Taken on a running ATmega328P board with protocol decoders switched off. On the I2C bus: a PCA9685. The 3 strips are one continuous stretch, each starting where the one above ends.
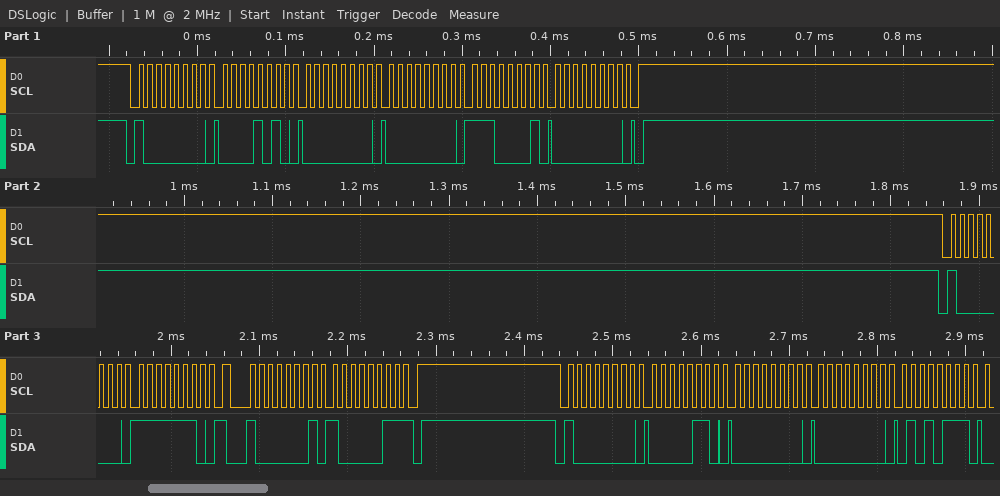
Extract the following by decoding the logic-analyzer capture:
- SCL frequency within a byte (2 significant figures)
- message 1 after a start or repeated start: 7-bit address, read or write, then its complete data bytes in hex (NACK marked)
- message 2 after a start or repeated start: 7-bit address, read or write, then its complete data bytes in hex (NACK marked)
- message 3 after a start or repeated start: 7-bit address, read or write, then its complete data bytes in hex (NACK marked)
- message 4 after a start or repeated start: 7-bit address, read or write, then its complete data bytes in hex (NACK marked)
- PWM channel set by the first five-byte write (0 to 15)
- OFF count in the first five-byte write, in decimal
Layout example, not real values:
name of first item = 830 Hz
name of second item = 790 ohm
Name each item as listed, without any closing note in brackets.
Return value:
SCL frequency within a byte = 100 kHz
message 1 after a start or repeated start: 7-bit address, read or write, then its complete data bytes in hex = 0x40 write: 0A 00 00 E1 00
message 2 after a start or repeated start: 7-bit address, read or write, then its complete data bytes in hex = 0x40 write: FE
message 3 after a start or repeated start: 7-bit address, read or write, then its complete data bytes in hex = 0x40 read: 83 NACK
message 4 after a start or repeated start: 7-bit address, read or write, then its complete data bytes in hex = 0x40 write: 06 00 00 57
PWM channel set by the first five-byte write = 1
OFF count in the first five-byte write, in decimal = 225
